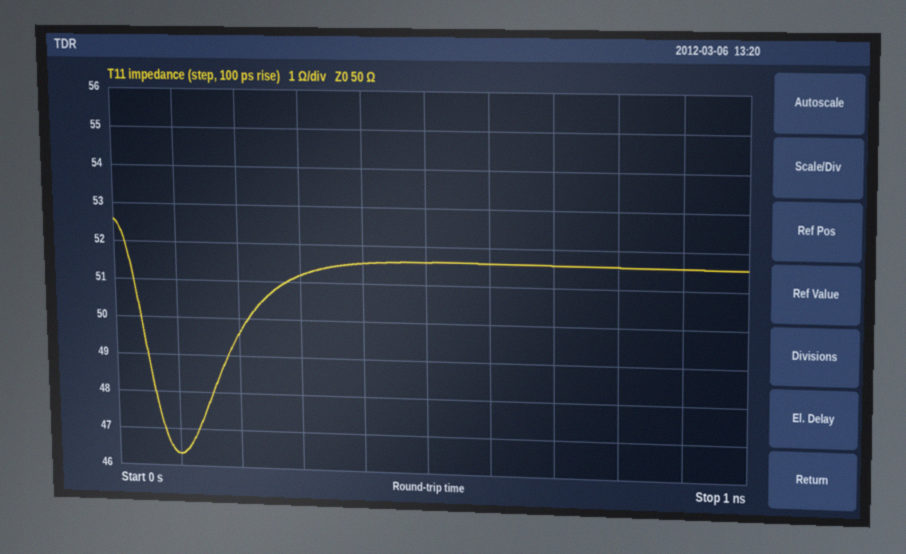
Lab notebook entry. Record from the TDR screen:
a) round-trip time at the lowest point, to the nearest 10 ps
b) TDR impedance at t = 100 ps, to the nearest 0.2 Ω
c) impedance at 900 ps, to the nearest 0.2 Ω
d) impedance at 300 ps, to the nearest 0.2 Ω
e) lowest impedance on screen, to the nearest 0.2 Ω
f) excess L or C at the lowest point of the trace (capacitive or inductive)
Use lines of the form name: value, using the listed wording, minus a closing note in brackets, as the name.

round-trip time at the lowest point, to the nearest 10 ps: 100 ps
TDR impedance at t = 100 ps, to the nearest 0.2 Ω: 46.4 Ω
impedance at 900 ps, to the nearest 0.2 Ω: 51.6 Ω
impedance at 300 ps, to the nearest 0.2 Ω: 51.2 Ω
lowest impedance on screen, to the nearest 0.2 Ω: 46.4 Ω
excess L or C at the lowest point of the trace: capacitive
